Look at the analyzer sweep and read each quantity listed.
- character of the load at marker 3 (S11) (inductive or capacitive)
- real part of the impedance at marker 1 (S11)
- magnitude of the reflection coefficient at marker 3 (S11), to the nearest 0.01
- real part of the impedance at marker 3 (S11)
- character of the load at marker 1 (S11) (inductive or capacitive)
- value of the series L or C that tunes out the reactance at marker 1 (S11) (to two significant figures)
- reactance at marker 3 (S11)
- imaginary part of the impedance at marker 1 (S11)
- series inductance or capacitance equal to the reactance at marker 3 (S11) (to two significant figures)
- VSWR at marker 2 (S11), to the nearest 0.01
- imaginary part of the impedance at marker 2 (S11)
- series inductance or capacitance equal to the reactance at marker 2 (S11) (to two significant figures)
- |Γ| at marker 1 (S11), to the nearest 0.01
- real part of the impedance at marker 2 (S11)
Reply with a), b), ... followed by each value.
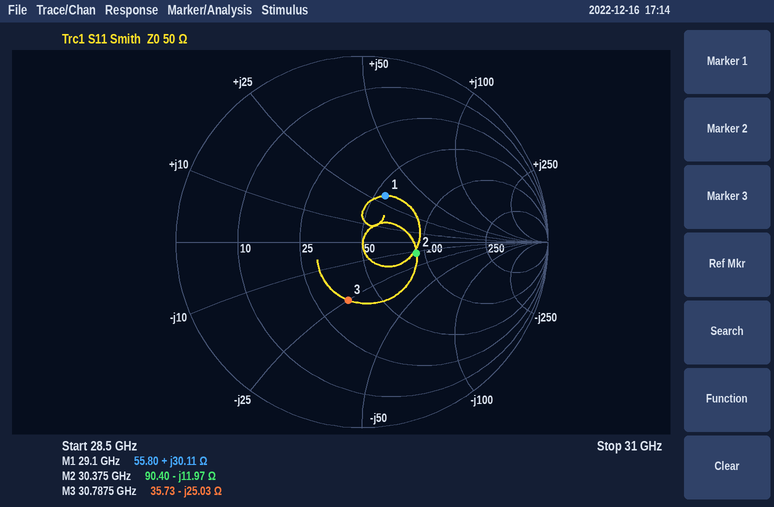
a) capacitive
b) 55.80 Ω
c) 0.32
d) 35.73 Ω
e) inductive
f) 180 fF
g) -25.03 Ω
h) +30.11 Ω
i) 210 fF
j) 1.85
k) -11.97 Ω
l) 440 fF
m) 0.28
n) 90.40 Ω
